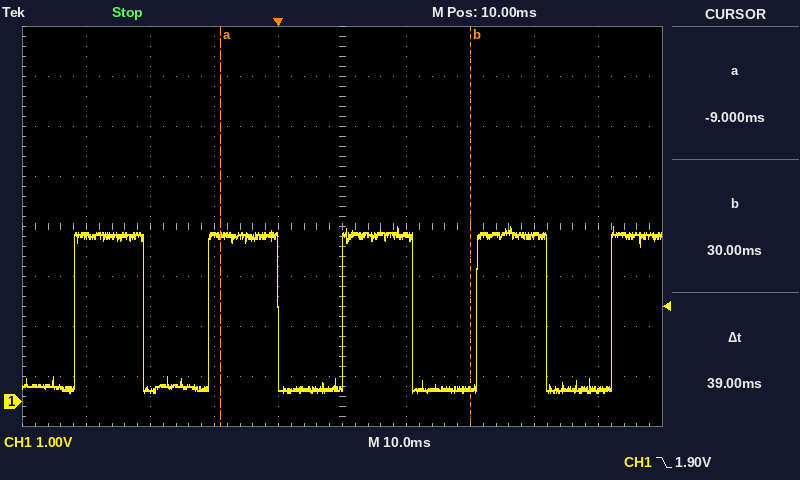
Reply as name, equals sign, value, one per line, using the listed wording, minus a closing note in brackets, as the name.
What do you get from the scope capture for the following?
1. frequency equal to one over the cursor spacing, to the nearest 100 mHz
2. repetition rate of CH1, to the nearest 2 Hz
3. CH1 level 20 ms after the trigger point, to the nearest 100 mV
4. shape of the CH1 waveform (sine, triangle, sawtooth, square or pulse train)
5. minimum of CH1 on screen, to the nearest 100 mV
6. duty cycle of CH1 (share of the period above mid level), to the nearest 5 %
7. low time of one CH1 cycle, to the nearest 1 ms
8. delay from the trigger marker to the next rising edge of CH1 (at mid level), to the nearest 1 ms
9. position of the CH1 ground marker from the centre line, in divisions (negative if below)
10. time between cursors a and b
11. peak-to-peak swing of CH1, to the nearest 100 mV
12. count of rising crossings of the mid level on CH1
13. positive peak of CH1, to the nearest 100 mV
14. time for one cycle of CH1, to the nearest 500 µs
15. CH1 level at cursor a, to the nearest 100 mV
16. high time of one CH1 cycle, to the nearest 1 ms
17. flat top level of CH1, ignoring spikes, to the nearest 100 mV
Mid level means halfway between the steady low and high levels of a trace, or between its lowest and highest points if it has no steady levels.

frequency equal to one over the cursor spacing, to the nearest 100 mHz = 25.6 Hz
repetition rate of CH1, to the nearest 2 Hz = 48 Hz
CH1 level 20 ms after the trigger point, to the nearest 100 mV = 3.3 V
shape of the CH1 waveform = square
minimum of CH1 on screen, to the nearest 100 mV = 200 mV
duty cycle of CH1 (share of the period above mid level), to the nearest 5 % = 50 %
low time of one CH1 cycle, to the nearest 1 ms = 10 ms
delay from the trigger marker to the next rising edge of CH1 (at mid level), to the nearest 1 ms = 10 ms
position of the CH1 ground marker from the centre line, in divisions = -3.5 div
time between cursors a and b = 39 ms
peak-to-peak swing of CH1, to the nearest 100 mV = 3.3 V
count of rising crossings of the mid level on CH1 = 5
positive peak of CH1, to the nearest 100 mV = 3.5 V
time for one cycle of CH1, to the nearest 500 µs = 21.0 ms
CH1 level at cursor a, to the nearest 100 mV = 3.3 V
high time of one CH1 cycle, to the nearest 1 ms = 11 ms
flat top level of CH1, ignoring spikes, to the nearest 100 mV = 3.3 V
